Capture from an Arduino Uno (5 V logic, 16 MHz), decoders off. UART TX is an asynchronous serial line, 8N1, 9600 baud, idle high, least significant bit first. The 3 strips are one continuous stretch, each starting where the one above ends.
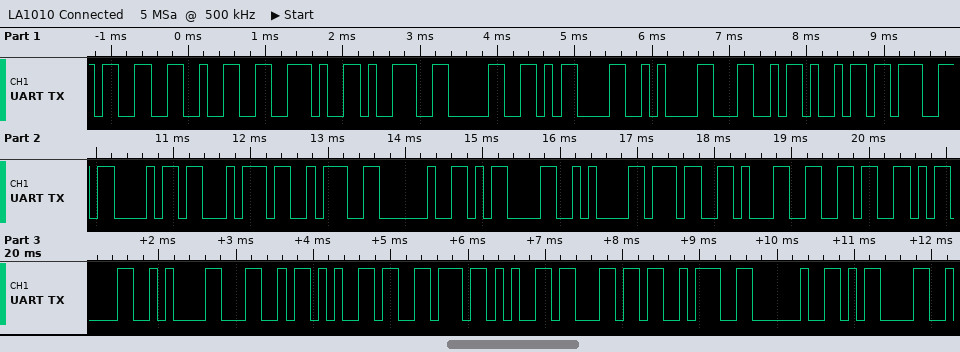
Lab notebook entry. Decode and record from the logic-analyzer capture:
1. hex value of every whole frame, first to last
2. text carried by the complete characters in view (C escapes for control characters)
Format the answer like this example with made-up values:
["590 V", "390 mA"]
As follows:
["33 32 2E 39 30 0D 0A 4C 69 67 68 74 3A 20 0D 0A 37 31 36 0D 0A 4C 65 76 65 6C 3A 20 0D", "\"32.90\\r\\nLight: \\r\\n716\\r\\nLevel: \\r\""]
